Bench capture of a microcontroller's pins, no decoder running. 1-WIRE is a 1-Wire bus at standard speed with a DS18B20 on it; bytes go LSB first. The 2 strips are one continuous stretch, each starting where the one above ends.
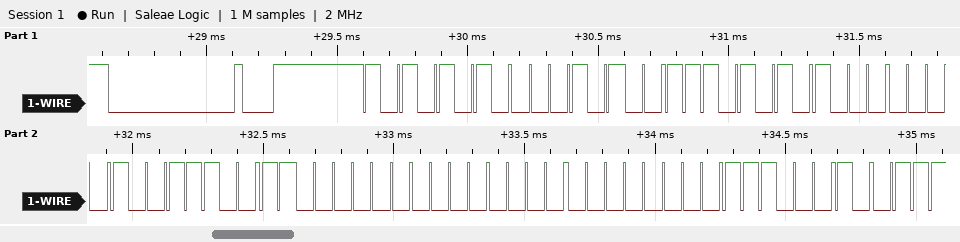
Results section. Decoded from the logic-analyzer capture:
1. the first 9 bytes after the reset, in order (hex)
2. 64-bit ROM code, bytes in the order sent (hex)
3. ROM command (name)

55 28 57 01 39 03 00 00 47
28 57 01 39 03 00 00 47
Match ROM
